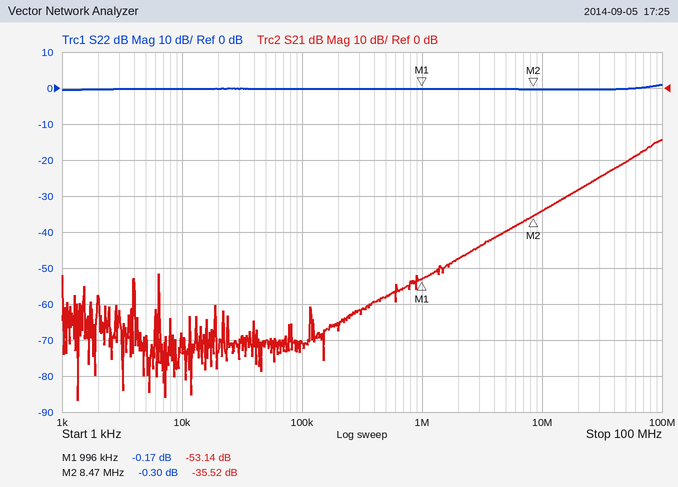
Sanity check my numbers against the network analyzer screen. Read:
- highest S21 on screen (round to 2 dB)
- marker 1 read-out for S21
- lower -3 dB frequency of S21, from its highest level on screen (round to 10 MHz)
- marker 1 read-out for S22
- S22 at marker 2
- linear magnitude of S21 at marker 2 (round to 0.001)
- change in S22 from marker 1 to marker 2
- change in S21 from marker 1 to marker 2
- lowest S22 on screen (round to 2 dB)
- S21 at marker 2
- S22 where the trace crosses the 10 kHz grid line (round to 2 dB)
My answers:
-14 dB
-53.14 dB
70 MHz
-0.17 dB
-0.30 dB
0.017
-0.13 dB
17.62 dB
0 dB
-35.52 dB
0 dB
